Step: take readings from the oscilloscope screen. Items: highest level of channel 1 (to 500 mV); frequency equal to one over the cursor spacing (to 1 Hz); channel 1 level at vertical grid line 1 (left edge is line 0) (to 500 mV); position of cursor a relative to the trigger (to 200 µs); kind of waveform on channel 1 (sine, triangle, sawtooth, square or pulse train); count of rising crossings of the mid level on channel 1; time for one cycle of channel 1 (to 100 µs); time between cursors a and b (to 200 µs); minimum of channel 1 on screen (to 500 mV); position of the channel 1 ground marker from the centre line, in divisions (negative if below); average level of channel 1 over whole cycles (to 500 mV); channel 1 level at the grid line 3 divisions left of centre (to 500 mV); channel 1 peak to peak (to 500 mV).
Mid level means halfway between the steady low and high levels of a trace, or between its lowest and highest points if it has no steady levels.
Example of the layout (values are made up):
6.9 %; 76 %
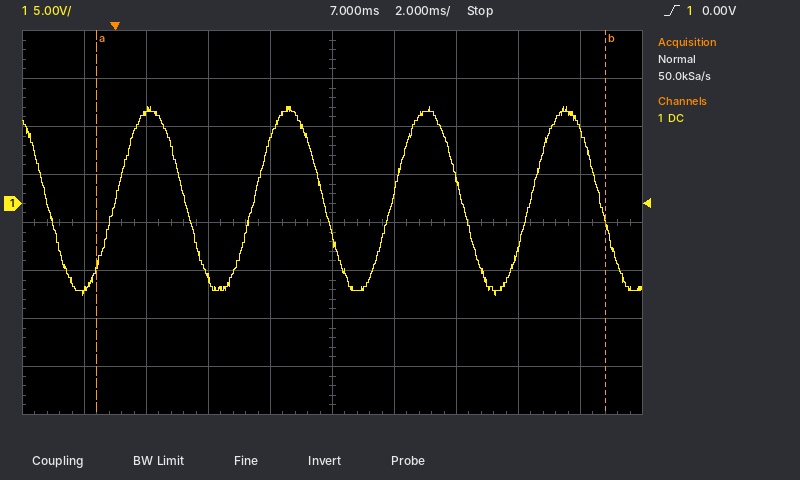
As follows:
10.0 V; 61 Hz; -9.0 V; -600 µs; sine; 4; 4.5 ms; 16.4 ms; -9.5 V; +0.4 div; 500 mV; 9.5 V; 19.5 V
